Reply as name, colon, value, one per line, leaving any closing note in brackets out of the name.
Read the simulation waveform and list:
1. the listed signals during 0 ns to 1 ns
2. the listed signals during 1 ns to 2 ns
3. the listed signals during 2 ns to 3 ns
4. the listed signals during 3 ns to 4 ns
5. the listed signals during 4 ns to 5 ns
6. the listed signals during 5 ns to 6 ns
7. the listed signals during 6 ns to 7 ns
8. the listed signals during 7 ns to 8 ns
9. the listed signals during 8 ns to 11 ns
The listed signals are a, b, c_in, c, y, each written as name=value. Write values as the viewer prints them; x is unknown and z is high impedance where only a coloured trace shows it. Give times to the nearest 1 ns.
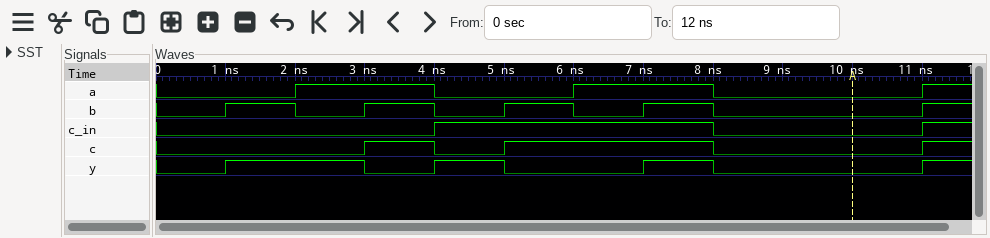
the listed signals during 0 ns to 1 ns: a=0, b=0, c_in=0, c=0, y=0
the listed signals during 1 ns to 2 ns: a=0, b=1, c_in=0, c=0, y=1
the listed signals during 2 ns to 3 ns: a=1, b=0, c_in=0, c=0, y=1
the listed signals during 3 ns to 4 ns: a=1, b=1, c_in=0, c=1, y=0
the listed signals during 4 ns to 5 ns: a=0, b=0, c_in=1, c=0, y=1
the listed signals during 5 ns to 6 ns: a=0, b=1, c_in=1, c=1, y=0
the listed signals during 6 ns to 7 ns: a=1, b=0, c_in=1, c=1, y=0
the listed signals during 7 ns to 8 ns: a=1, b=1, c_in=1, c=1, y=1
the listed signals during 8 ns to 11 ns: a=0, b=0, c_in=0, c=0, y=0
